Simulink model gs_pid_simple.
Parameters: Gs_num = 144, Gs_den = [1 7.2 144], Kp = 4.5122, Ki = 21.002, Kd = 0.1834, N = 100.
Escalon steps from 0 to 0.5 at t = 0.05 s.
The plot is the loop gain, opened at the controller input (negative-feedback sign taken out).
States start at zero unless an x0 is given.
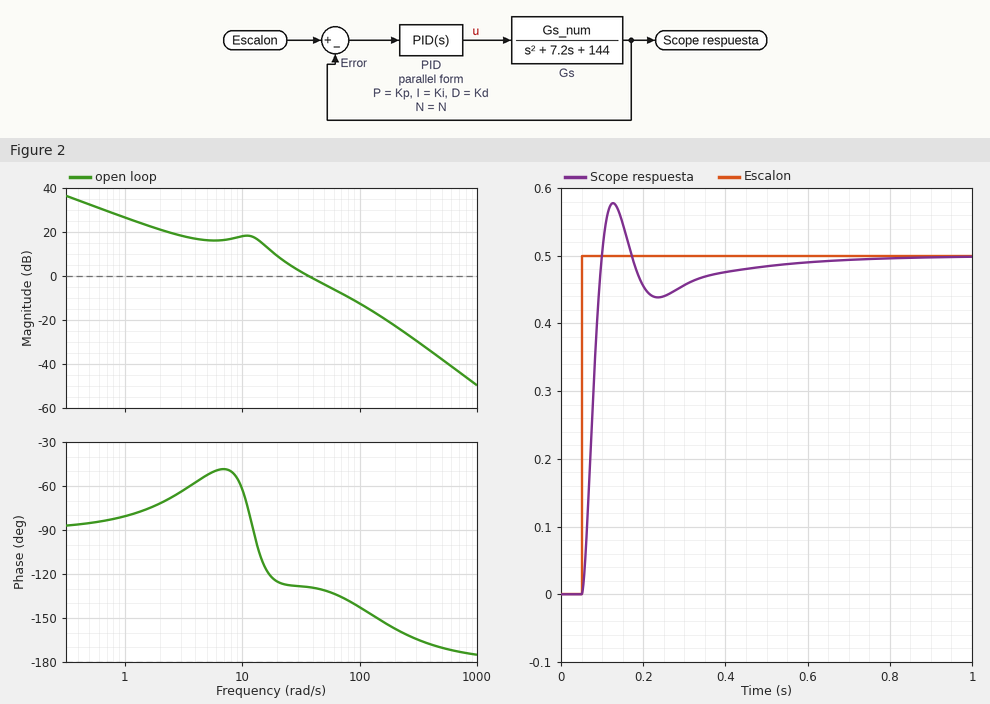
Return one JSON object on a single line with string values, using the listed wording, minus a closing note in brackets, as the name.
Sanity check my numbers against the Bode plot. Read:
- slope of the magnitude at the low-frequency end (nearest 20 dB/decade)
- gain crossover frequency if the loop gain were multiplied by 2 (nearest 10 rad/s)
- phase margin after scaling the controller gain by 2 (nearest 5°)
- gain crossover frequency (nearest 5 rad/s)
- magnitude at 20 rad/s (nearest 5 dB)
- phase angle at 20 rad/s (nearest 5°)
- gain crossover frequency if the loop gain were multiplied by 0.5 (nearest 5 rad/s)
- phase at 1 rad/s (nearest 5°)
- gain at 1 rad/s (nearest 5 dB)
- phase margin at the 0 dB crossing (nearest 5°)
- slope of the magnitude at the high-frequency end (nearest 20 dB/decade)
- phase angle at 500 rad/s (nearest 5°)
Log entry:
{"slope of the magnitude at the low-frequency end": "-20 dB/decade", "gain crossover frequency if the loop gain were multiplied by 2": "60 rad/s", "phase margin after scaling the controller gain by 2": "45°", "gain crossover frequency": "35 rad/s", "magnitude at 20 rad/s": "10 dB", "phase angle at 20 rad/s": "-125°", "gain crossover frequency if the loop gain were multiplied by 0.5": "25 rad/s", "phase at 1 rad/s": "-80°", "gain at 1 rad/s": "25 dB", "phase margin at the 0 dB crossing": "50°", "slope of the magnitude at the high-frequency end": "-40 dB/decade", "phase angle at 500 rad/s": "-170°"}
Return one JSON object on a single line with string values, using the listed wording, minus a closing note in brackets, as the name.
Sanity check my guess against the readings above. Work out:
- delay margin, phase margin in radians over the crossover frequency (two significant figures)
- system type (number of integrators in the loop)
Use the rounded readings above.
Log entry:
{"delay margin, phase margin in radians over the crossover frequency": "0.025 s", "system type": "1"}
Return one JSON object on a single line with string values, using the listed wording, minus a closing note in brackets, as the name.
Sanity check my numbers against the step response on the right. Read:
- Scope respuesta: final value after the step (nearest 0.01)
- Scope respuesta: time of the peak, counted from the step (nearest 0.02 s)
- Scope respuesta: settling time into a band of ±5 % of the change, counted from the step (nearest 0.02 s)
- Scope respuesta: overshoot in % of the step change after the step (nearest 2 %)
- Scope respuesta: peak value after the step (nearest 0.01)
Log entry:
{"Scope respuesta: final value after the step": "0.50", "Scope respuesta: time of the peak, counted from the step": "0.08 s", "Scope respuesta: settling time into a band of ±5 % of the change, counted from the step": "0.34 s", "Scope respuesta: overshoot in % of the step change after the step": "16 %", "Scope respuesta: peak value after the step": "0.58"}
